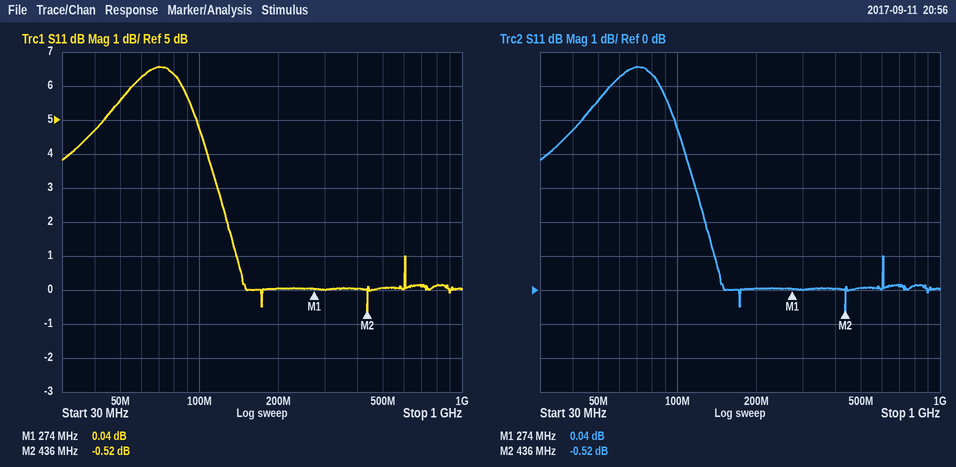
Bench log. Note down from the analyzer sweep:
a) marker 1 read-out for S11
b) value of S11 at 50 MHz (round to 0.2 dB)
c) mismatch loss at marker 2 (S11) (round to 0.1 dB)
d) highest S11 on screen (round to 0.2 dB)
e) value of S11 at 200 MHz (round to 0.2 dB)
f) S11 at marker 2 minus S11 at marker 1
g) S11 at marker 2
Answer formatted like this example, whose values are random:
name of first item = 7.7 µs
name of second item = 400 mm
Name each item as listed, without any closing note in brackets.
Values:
marker 1 read-out for S11 = 0.04 dB
value of S11 at 50 MHz = 5.6 dB
mismatch loss at marker 2 (S11) = 9.5 dB
highest S11 on screen = 6.6 dB
value of S11 at 200 MHz = 0.0 dB
S11 at marker 2 minus S11 at marker 1 = -0.56 dB
S11 at marker 2 = -0.52 dB
